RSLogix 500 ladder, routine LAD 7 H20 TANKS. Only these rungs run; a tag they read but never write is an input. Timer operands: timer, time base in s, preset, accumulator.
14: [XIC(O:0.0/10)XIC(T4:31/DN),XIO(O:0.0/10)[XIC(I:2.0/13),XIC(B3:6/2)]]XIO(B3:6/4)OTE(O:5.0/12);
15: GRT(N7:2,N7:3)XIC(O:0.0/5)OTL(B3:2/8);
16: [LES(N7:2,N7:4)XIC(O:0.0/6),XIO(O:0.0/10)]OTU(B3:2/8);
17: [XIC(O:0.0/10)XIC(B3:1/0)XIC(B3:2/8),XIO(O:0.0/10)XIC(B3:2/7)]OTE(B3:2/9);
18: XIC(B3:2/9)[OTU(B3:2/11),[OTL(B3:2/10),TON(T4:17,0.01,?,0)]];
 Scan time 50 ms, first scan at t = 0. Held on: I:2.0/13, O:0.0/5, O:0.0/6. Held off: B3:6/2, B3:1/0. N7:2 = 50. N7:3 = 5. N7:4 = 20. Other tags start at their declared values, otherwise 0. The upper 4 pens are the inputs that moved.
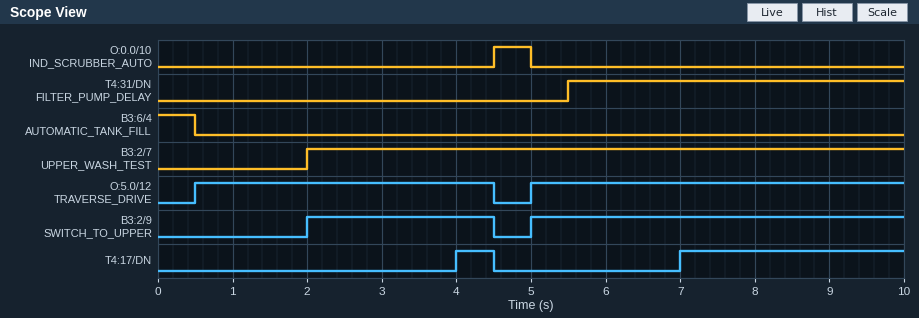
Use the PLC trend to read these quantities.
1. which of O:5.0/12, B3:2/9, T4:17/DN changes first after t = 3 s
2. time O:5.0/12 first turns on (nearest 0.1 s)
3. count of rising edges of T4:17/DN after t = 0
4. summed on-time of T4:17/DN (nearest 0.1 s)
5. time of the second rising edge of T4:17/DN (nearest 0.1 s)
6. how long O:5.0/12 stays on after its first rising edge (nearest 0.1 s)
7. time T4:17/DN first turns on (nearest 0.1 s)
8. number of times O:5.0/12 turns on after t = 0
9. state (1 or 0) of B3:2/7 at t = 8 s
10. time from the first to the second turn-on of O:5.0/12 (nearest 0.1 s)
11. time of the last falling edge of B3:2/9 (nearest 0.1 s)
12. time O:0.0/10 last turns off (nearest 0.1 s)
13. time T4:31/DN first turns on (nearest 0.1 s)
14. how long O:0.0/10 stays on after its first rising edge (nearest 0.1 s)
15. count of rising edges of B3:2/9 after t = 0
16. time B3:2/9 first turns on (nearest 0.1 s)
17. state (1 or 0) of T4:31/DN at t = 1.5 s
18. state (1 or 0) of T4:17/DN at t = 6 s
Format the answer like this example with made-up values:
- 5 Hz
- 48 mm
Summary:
- T4:17/DN
- 0.5 s
- 2
- 3.5 s
- 7.0 s
- 4.0 s
- 4.0 s
- 2
- 1
- 4.5 s
- 4.5 s
- 5.0 s
- 5.5 s
- 0.5 s
- 2
- 2.0 s
- 0
- 0
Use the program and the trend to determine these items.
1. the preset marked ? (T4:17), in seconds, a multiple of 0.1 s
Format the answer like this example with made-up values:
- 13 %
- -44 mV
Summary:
- 2.0 s
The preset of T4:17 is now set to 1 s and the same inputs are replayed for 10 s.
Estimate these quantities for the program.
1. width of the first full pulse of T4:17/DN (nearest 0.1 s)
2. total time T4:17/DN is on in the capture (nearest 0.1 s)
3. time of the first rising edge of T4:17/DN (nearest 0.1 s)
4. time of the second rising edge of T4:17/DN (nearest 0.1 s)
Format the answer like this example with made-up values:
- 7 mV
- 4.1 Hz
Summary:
- 1.5 s
- 5.5 s
- 3.0 s
- 6.0 s
